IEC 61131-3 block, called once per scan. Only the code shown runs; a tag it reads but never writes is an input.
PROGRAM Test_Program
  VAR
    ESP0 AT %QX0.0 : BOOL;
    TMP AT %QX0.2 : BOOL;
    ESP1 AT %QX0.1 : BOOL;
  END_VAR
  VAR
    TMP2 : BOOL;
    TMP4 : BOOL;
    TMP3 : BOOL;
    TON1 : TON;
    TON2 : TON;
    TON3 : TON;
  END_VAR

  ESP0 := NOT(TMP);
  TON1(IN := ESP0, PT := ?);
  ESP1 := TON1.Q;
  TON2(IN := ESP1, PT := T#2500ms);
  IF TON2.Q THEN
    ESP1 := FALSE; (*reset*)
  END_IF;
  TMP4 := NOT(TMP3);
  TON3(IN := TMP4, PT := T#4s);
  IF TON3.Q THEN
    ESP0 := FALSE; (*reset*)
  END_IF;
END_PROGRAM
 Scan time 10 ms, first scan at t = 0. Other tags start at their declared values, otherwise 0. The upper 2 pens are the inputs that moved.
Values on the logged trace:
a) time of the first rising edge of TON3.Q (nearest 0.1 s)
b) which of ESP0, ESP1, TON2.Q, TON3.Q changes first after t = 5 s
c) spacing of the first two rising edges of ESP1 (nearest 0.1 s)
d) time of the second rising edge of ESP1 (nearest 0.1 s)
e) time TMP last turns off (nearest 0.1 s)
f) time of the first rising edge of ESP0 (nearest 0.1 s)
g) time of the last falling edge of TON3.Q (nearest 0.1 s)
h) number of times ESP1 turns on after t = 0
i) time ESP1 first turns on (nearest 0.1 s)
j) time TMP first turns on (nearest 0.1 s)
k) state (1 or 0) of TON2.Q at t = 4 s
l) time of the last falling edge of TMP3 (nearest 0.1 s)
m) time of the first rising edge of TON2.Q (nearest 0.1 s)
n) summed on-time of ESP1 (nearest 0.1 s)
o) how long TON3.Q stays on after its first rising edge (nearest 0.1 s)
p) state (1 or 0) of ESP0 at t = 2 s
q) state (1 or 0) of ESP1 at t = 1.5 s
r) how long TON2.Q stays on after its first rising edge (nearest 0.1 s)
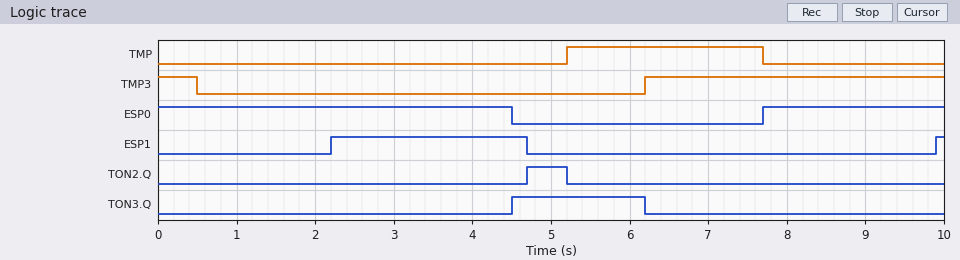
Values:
4.5 s
TON2.Q
7.7 s
9.9 s
7.7 s
7.7 s
6.2 s
2
2.2 s
5.2 s
0
0.5 s
4.7 s
2.6 s
1.7 s
1
0
0.5 s
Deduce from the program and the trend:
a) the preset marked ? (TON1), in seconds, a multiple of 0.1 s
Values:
2.2 s
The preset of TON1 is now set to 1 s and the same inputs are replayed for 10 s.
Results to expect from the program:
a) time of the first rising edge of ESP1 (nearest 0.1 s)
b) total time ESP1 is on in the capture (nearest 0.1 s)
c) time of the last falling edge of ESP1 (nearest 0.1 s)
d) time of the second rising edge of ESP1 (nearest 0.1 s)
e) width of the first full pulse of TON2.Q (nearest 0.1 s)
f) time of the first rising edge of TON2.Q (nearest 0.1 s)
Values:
1.0 s
3.8 s
3.5 s
8.7 s
1.7 s
3.5 s
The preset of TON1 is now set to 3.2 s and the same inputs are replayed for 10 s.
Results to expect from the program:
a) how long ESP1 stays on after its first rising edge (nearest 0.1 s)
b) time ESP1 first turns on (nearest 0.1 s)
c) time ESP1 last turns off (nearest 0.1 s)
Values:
2.0 s
3.2 s
5.2 s
